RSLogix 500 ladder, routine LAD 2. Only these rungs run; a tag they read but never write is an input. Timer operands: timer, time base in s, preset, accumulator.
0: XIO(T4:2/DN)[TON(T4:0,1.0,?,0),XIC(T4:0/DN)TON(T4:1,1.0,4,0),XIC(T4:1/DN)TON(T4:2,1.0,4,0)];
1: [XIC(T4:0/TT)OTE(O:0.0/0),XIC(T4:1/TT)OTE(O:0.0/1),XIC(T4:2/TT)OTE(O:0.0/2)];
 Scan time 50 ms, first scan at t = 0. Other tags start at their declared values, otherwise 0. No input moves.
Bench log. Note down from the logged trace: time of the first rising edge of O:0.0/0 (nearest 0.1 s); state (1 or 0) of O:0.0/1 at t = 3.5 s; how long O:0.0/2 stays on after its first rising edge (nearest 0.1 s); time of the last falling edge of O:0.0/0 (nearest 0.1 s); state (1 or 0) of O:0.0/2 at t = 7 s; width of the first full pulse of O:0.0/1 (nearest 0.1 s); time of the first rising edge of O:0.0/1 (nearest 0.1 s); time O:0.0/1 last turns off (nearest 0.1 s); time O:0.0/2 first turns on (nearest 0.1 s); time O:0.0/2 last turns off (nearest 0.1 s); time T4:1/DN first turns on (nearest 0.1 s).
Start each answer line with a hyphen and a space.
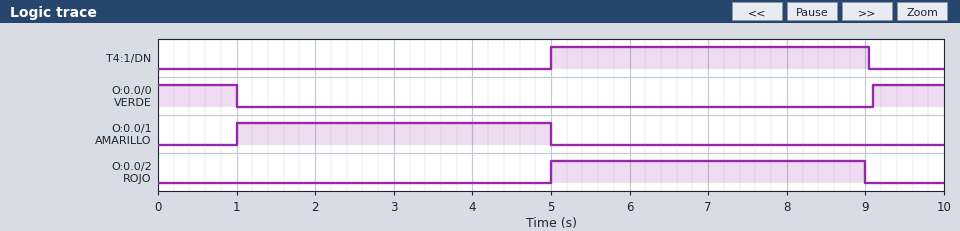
- 9.1 s
- 1
- 4.0 s
- 1.0 s
- 1
- 4.0 s
- 1.0 s
- 5.0 s
- 5.0 s
- 9.0 s
- 5.0 s
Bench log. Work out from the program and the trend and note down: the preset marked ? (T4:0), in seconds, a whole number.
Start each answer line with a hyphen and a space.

- 1 s
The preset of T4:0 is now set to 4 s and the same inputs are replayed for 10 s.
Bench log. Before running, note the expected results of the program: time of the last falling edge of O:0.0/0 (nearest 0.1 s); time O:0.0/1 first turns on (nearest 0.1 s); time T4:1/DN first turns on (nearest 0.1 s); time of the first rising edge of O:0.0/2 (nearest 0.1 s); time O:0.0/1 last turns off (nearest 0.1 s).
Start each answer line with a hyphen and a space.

- 4.0 s
- 4.0 s
- 8.0 s
- 8.0 s
- 8.0 s
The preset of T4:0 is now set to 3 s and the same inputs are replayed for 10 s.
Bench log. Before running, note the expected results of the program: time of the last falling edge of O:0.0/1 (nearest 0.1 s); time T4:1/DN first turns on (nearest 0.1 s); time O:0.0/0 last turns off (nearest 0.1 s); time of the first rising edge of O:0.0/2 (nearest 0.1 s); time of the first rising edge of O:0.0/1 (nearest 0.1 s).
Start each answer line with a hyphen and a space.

- 7.0 s
- 7.0 s
- 3.0 s
- 7.0 s
- 3.0 s
